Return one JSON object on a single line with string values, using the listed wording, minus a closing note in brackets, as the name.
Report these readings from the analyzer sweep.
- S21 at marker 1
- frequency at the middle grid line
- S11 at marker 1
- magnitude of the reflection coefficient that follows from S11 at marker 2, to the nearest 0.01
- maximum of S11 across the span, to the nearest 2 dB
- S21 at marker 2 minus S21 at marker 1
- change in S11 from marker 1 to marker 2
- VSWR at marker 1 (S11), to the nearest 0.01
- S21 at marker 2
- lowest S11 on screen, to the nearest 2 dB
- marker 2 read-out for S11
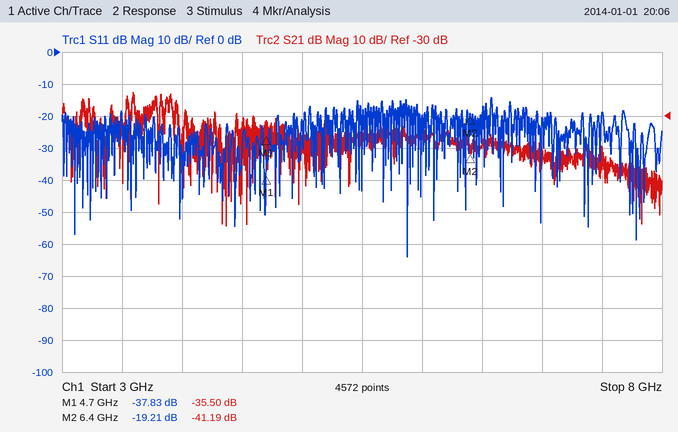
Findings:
{"S21 at marker 1": "-35.50 dB", "frequency at the middle grid line": "5.5 GHz", "S11 at marker 1": "-37.83 dB", "magnitude of the reflection coefficient that follows from S11 at marker 2, to the nearest 0.01": "0.11", "maximum of S11 across the span, to the nearest 2 dB": "-14 dB", "S21 at marker 2 minus S21 at marker 1": "-5.69 dB", "change in S11 from marker 1 to marker 2": "18.62 dB", "VSWR at marker 1 (S11), to the nearest 0.01": "1.03", "S21 at marker 2": "-41.19 dB", "lowest S11 on screen, to the nearest 2 dB": "-64 dB", "marker 2 read-out for S11": "-19.21 dB"}
